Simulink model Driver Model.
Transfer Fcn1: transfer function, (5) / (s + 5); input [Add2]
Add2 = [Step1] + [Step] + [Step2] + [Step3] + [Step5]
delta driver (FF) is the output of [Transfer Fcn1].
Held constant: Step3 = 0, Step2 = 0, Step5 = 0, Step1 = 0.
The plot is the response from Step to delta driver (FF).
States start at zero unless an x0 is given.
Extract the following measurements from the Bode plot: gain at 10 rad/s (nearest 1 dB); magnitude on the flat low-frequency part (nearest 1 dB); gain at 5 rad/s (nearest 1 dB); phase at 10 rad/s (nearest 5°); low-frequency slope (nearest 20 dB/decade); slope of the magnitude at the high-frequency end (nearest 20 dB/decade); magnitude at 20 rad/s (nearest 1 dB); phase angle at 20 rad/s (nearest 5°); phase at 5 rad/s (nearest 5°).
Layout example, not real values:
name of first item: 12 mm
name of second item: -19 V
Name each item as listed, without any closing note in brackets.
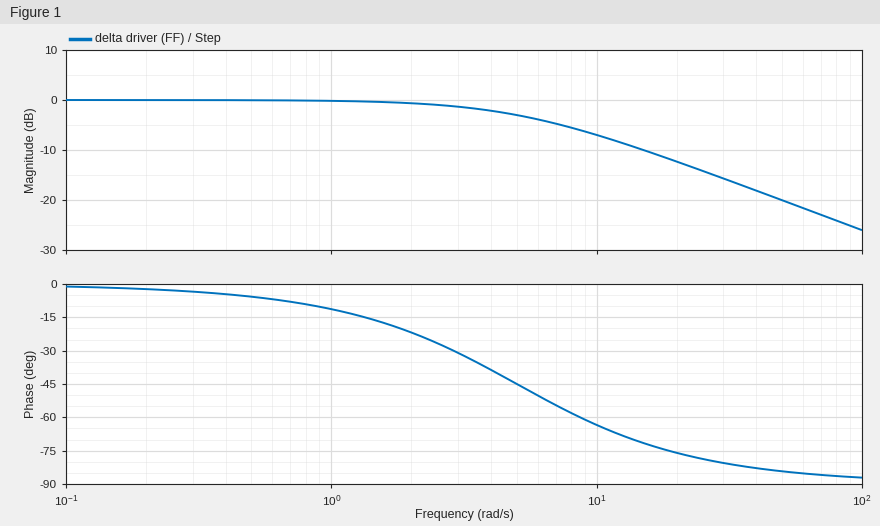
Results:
gain at 10 rad/s: -7 dB
magnitude on the flat low-frequency part: 0 dB
gain at 5 rad/s: -3 dB
phase at 10 rad/s: -65°
low-frequency slope: 0 dB/decade
slope of the magnitude at the high-frequency end: -20 dB/decade
magnitude at 20 rad/s: -12 dB
phase angle at 20 rad/s: -75°
phase at 5 rad/s: -45°
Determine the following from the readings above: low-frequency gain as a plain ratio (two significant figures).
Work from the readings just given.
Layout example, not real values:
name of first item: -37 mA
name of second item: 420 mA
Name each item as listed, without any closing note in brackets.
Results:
low-frequency gain as a plain ratio: 1.0
